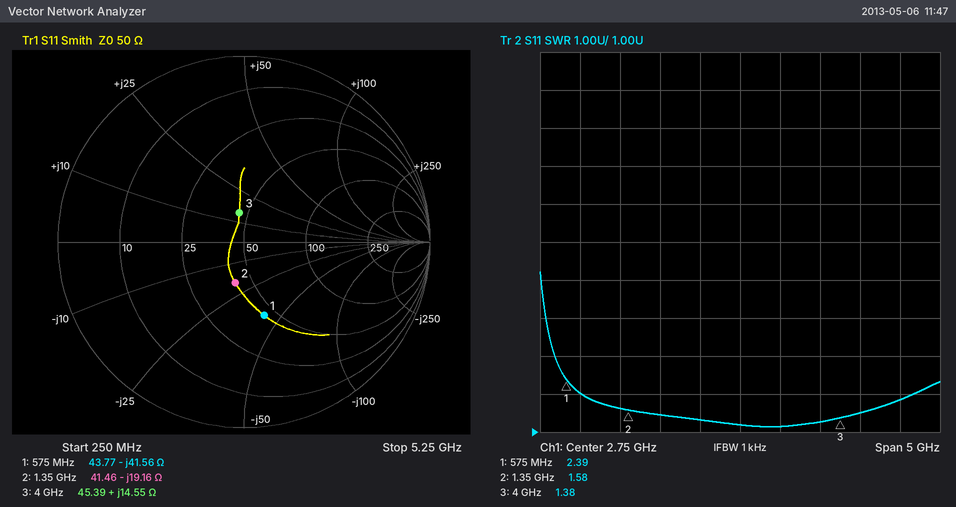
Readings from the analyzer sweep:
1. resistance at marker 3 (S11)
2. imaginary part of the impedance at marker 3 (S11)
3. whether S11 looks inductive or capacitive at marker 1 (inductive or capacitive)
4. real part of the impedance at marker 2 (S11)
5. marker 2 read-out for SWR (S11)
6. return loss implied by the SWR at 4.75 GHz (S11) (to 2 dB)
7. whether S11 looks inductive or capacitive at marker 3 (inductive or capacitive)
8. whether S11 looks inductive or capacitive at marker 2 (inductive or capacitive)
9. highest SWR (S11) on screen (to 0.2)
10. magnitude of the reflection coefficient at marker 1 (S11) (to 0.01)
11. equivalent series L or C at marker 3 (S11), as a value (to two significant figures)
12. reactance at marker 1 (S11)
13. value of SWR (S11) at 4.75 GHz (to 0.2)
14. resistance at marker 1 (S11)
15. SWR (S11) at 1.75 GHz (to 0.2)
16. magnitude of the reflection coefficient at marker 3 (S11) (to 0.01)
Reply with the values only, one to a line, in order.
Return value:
45.39 Ω
+14.55 Ω
capacitive
41.46 Ω
1.58
10 dB
inductive
capacitive
5.2
0.41
580 pH
-41.56 Ω
1.8
43.77 Ω
1.4
0.16
